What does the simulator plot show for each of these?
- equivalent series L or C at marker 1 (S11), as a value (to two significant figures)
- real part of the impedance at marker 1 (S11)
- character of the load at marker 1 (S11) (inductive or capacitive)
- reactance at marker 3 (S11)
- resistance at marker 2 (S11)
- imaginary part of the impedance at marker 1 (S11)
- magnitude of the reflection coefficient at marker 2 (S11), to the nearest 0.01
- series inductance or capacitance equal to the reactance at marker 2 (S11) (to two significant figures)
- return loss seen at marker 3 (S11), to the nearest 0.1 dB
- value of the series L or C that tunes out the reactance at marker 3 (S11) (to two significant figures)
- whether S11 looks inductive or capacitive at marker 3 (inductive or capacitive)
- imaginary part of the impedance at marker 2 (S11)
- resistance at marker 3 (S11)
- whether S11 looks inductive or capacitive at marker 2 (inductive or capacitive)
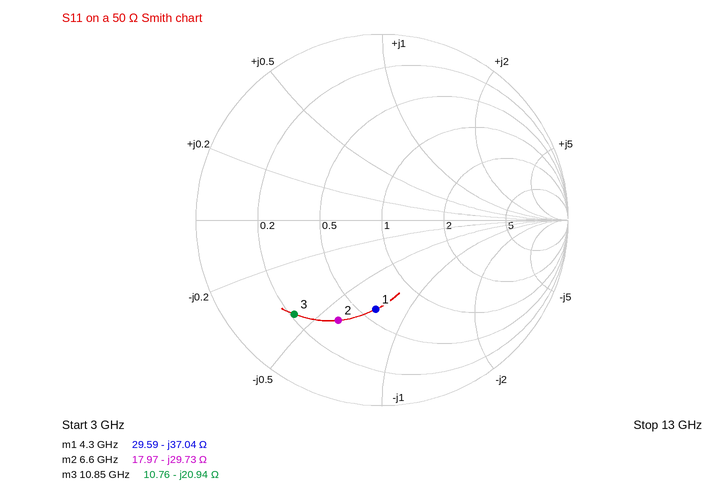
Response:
1.00 pF
29.59 Ω
capacitive
-20.94 Ω
17.97 Ω
-37.04 Ω
0.59
810 fF
3.2 dB
310 pH
capacitive
-29.73 Ω
10.76 Ω
capacitive
